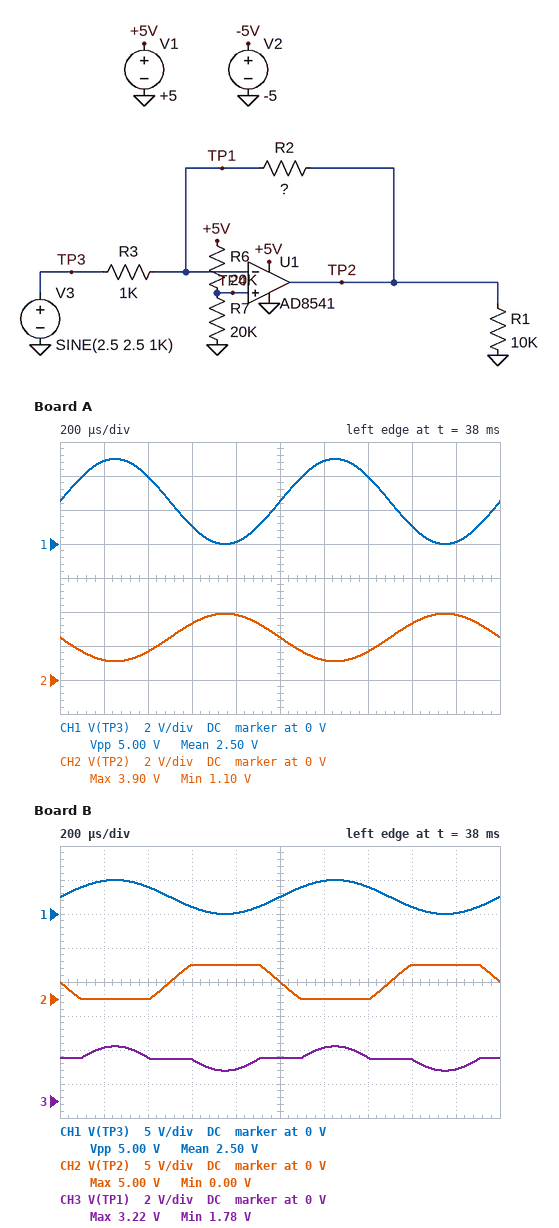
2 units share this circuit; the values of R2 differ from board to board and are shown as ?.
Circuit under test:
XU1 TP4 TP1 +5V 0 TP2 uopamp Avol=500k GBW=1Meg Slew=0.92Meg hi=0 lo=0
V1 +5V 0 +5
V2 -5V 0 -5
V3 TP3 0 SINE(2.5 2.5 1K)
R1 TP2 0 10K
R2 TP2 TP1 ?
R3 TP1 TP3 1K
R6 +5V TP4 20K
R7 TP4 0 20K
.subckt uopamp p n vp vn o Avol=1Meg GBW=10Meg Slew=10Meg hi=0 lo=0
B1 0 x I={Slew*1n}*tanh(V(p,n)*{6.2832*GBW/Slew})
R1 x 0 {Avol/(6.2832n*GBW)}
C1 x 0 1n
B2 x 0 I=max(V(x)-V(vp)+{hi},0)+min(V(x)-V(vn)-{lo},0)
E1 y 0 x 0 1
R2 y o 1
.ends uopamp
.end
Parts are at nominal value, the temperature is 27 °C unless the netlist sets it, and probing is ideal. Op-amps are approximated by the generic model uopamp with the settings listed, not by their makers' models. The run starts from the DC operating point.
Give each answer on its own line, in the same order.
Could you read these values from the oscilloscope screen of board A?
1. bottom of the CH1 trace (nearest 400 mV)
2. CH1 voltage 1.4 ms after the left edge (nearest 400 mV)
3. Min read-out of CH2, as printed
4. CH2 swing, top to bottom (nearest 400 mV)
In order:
0 V
4.0 V
1.10 V
2.8 V
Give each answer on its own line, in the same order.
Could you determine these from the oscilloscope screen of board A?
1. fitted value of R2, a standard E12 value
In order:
560 Ω
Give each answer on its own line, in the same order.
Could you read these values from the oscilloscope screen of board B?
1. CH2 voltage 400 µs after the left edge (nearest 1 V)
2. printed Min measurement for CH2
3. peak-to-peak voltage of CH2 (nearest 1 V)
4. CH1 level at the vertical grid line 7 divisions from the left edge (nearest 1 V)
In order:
0 V
0.00 V
5 V
4 V
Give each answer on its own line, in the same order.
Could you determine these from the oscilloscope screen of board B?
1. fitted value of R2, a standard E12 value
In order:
1.8 kΩ
